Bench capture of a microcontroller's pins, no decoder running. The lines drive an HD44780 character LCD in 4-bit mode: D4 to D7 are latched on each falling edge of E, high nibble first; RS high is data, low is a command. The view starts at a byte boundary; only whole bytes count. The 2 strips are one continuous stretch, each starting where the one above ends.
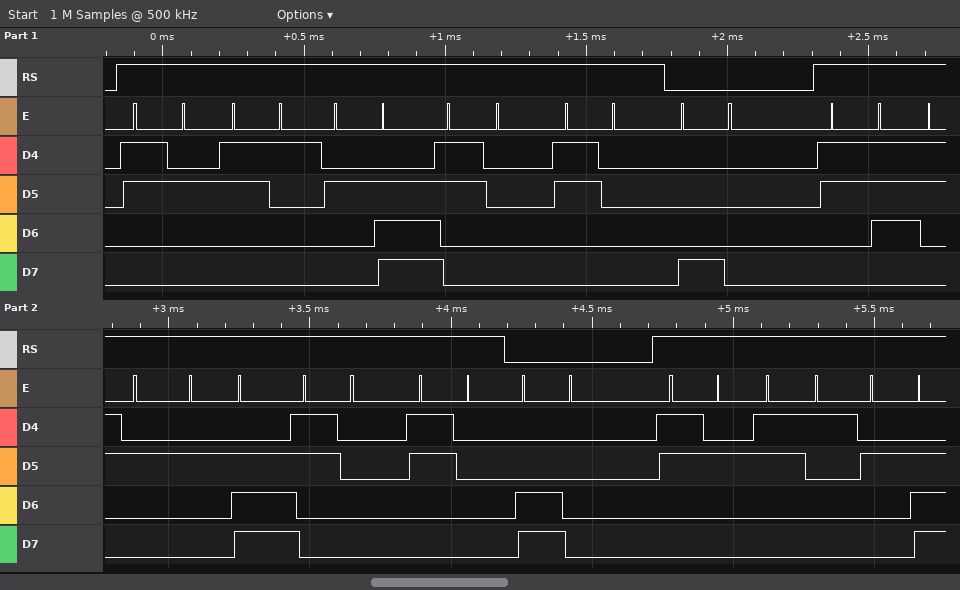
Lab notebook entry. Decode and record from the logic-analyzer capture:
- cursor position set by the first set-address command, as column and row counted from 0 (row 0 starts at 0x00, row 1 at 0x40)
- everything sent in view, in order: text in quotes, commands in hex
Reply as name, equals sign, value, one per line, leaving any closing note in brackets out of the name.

cursor position set by the first set-address command, as column and row counted from 0 = column 0, row 0
everything sent in view, in order: text in quotes, commands in hex = "21.00" 0x80 "72.00" 0xC0 "21."
